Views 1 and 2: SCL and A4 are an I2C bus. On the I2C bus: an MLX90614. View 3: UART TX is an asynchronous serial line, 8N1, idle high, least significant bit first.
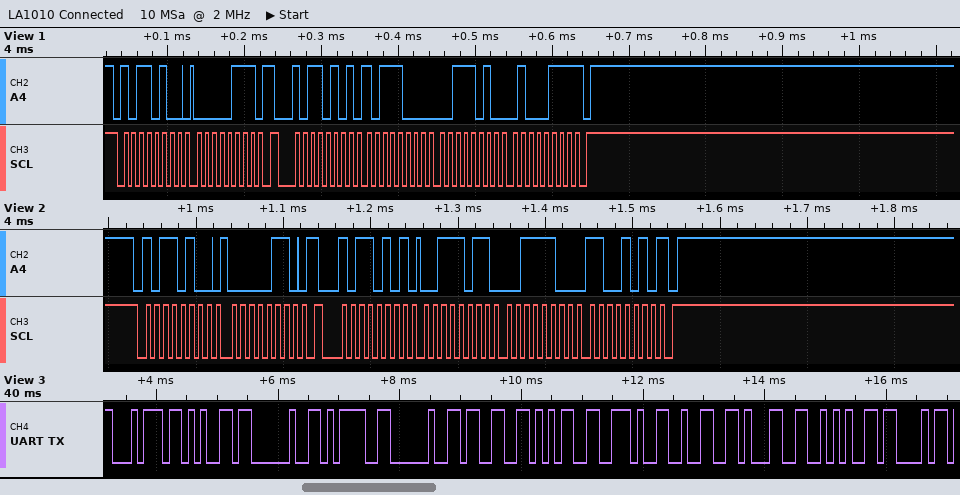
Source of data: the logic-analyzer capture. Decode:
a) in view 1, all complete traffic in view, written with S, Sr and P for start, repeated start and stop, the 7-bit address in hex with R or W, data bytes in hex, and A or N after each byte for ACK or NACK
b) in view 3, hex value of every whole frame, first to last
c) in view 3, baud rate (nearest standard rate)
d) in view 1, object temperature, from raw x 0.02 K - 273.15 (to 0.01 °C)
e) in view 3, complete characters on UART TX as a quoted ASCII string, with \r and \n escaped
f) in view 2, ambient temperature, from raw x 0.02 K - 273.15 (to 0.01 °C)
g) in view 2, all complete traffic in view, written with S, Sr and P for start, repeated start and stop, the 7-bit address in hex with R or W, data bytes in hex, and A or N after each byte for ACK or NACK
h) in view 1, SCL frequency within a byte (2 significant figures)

S 5AW A 07 A Sr 5AR A B8 A 3A A 47 N P
0x74 0x65 0x20 0x3D 0x20 0x33 0x35 0x2E 0x32 0x31 0x2A 0x43
9600 baud
27.49 °C
"te = 35.21*C"
35.23 °C
S 5AW A 06 A Sr 5AR A 3B A 3C A CA N P
100 kHz
